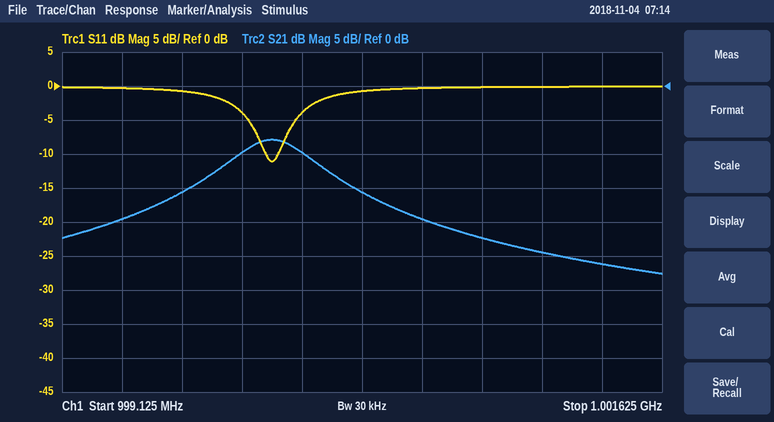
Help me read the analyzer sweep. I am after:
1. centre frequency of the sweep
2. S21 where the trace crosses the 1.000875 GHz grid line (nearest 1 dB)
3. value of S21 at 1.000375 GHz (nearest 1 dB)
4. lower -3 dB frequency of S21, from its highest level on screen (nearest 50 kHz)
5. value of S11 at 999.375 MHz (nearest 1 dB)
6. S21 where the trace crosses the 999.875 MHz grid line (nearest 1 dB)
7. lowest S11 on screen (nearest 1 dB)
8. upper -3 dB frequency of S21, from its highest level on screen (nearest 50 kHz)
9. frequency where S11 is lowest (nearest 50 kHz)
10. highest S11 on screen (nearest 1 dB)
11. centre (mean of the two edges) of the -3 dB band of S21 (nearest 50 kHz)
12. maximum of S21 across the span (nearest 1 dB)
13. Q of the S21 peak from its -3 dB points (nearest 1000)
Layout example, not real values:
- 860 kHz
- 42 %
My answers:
- 1.000375 GHz
- -22 dB
- -16 dB
- 999.85 MHz
- 0 dB
- -10 dB
- -11 dB
- 1.00015 GHz
- 1.00000 GHz
- 0 dB
- 1.00000 GHz
- -8 dB
- 3000
